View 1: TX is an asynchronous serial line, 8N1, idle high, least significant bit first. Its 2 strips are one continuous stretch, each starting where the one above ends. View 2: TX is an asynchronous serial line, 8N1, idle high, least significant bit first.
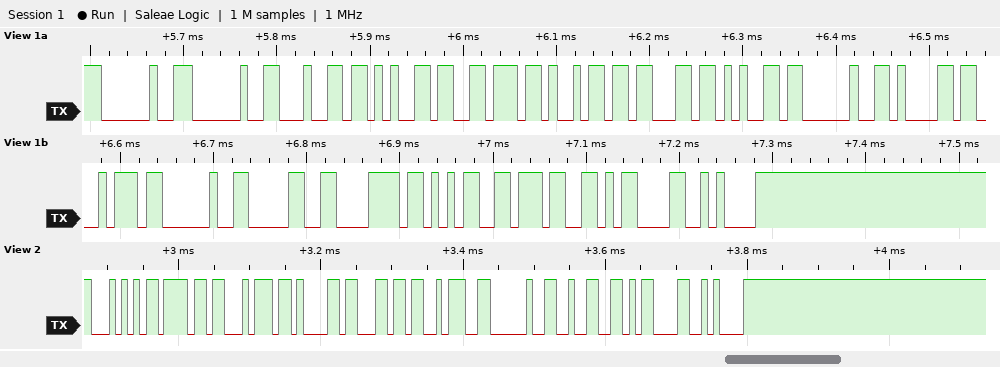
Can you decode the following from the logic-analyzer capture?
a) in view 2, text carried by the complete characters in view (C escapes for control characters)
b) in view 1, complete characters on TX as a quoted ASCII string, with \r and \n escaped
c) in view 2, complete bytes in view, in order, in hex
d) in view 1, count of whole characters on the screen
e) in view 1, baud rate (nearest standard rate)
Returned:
"Total: 2\r\n"
"  device at 0x57\r\n"
54 6F 74 61 6C 3A 20 32 0D 0A
18
115200 baud
